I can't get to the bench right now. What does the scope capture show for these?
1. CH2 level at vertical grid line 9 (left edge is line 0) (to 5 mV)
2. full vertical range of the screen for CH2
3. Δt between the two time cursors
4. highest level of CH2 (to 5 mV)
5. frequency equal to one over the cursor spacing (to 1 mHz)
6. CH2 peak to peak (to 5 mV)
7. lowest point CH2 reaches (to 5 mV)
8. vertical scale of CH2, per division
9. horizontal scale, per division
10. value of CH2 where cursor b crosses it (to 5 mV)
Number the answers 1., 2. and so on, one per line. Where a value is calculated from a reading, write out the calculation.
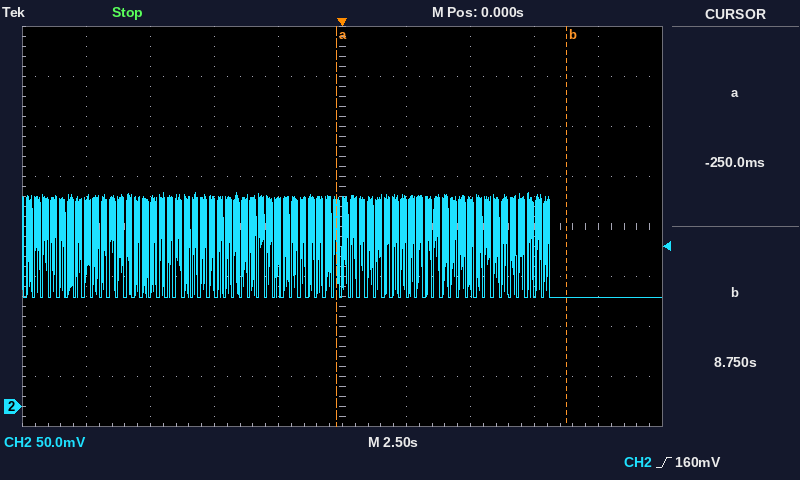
1. 110 mV
2. 400 mV
3. 8.75 s − (-250 ms) = 9.00 s
4. 215 mV
5. 1 / 9.00 s ≈ 111 mHz
6. 215 mV − (110 mV) = 105 mV
7. 110 mV
8. 50 mV
9. 2.5 s
10. 110 mV
